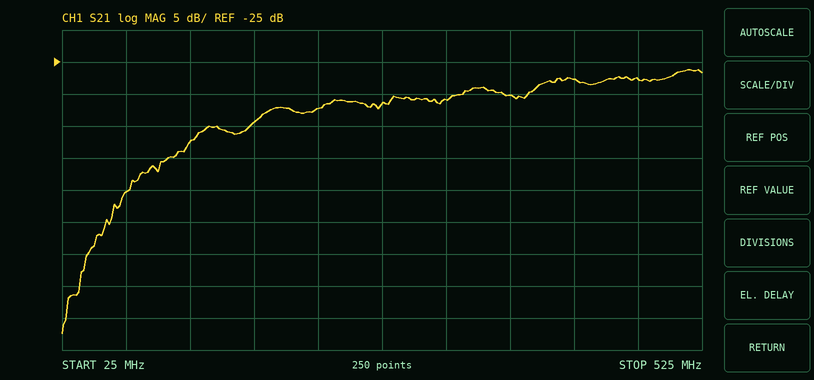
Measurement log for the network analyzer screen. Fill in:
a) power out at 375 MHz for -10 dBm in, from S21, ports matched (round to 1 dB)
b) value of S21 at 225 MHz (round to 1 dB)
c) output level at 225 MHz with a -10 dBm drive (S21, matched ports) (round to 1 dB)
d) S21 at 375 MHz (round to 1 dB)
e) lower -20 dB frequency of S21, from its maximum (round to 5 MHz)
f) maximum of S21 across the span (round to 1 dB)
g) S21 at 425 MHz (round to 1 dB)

-40 dBm
-32 dB
-42 dBm
-30 dB
70 MHz
-26 dB
-28 dB
